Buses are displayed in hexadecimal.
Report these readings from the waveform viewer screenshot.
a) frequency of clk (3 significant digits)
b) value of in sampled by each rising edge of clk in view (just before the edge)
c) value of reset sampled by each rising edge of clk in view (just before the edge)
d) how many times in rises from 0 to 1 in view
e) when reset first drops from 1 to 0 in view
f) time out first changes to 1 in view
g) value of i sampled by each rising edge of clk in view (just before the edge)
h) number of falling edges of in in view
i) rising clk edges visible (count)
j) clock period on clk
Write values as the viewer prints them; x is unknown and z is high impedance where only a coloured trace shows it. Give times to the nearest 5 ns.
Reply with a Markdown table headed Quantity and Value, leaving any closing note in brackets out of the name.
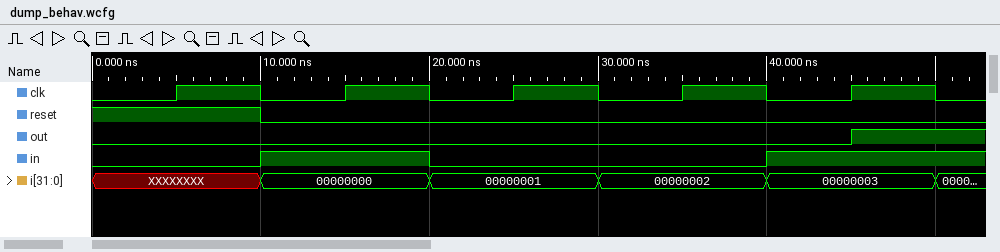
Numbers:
| Quantity | Value |
|---|---|
| frequency of clk | 100 MHz |
| value of in sampled by each rising edge of clk in view | 0 1 0 0 1 |
| value of reset sampled by each rising edge of clk in view | 1 0 0 0 0 |
| how many times in rises from 0 to 1 in view | 2 |
| when reset first drops from 1 to 0 in view | 10 ns |
| time out first changes to 1 in view | 45 ns |
| value of i sampled by each rising edge of clk in view | XXXXXXXX, 00000000, 00000001, 00000002, 00000003 |
| number of falling edges of in in view | 1 |
| rising clk edges visible | 5 |
| clock period on clk | 10 ns |
